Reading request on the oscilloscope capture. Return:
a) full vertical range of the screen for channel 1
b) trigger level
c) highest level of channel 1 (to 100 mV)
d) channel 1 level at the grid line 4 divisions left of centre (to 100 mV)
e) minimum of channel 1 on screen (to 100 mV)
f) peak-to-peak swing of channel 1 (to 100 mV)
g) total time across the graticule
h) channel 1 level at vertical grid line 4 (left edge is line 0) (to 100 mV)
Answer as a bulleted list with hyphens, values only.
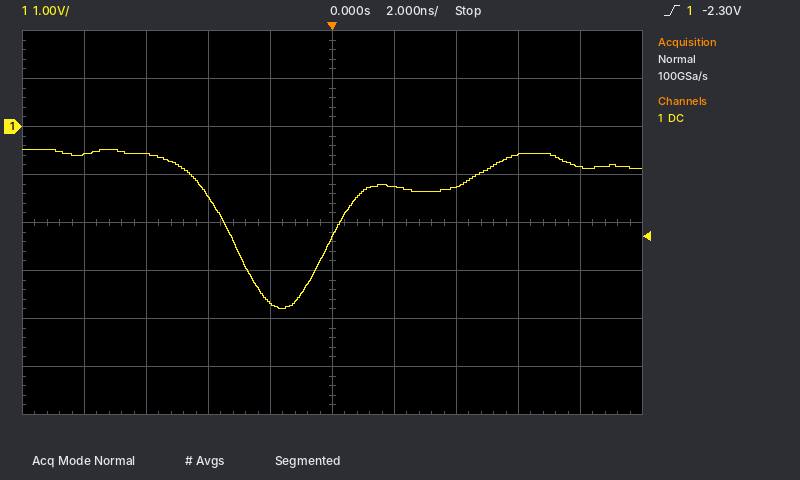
- 8 V
- -2.30 V
- -500 mV
- -600 mV
- -3.8 V
- 3.3 V
- 20 ns
- -3.7 V
